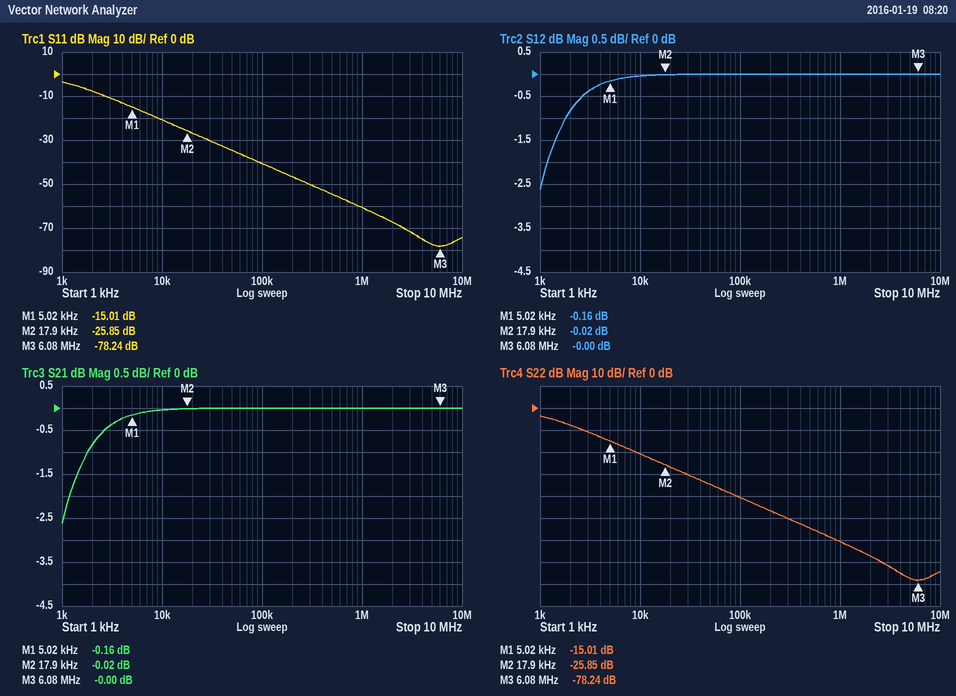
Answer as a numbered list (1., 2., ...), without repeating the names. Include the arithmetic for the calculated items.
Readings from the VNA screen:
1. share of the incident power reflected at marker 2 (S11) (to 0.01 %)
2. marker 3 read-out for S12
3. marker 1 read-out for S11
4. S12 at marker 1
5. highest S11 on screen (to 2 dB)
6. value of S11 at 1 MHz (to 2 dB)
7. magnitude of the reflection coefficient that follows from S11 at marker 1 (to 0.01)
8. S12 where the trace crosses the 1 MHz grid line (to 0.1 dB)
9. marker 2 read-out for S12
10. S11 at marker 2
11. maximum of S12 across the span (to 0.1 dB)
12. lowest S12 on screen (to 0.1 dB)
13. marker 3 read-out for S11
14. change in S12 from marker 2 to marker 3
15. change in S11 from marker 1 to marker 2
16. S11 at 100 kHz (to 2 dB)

1. 10^(-25.85/10) ≈ 0.26 %
2. -0.00 dB
3. -15.01 dB
4. -0.16 dB
5. -4 dB
6. -60 dB
7. 10^(-15.01/20) ≈ 0.18
8. 0.0 dB
9. -0.02 dB
10. -25.85 dB
11. 0.0 dB
12. -2.6 dB
13. -78.24 dB
14. -0 − (-0.02) = 0.02 dB
15. -25.85 − (-15.01) = -10.84 dB
16. -40 dB
